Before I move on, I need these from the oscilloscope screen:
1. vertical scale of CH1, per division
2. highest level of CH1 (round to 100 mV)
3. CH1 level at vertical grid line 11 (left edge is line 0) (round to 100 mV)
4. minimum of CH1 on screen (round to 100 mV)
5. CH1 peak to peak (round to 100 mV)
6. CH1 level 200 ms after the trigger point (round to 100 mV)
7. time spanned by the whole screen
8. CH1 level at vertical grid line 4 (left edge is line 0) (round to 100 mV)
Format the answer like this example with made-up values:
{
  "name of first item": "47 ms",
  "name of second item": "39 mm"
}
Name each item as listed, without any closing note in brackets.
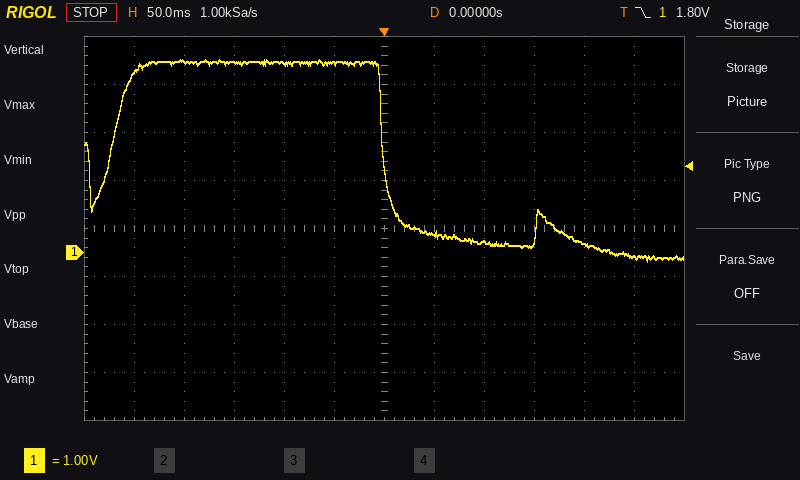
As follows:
{
  "vertical scale of CH1, per division": "1 V",
  "highest level of CH1": "4.0 V",
  "CH1 level at vertical grid line 11 (left edge is line 0)": "-100 mV",
  "minimum of CH1 on screen": "-200 mV",
  "CH1 peak to peak": "4.2 V",
  "CH1 level 200 ms after the trigger point": "200 mV",
  "time spanned by the whole screen": "600 ms",
  "CH1 level at vertical grid line 4 (left edge is line 0)": "3.9 V"
}
